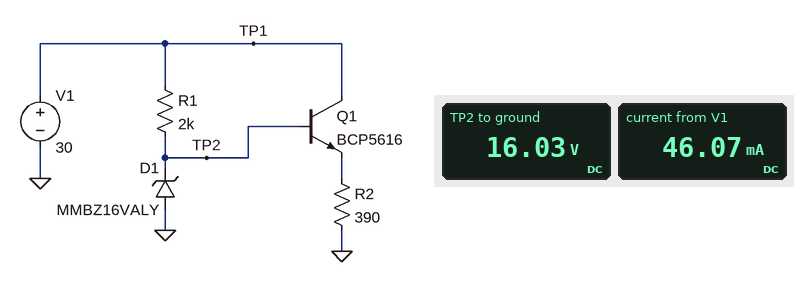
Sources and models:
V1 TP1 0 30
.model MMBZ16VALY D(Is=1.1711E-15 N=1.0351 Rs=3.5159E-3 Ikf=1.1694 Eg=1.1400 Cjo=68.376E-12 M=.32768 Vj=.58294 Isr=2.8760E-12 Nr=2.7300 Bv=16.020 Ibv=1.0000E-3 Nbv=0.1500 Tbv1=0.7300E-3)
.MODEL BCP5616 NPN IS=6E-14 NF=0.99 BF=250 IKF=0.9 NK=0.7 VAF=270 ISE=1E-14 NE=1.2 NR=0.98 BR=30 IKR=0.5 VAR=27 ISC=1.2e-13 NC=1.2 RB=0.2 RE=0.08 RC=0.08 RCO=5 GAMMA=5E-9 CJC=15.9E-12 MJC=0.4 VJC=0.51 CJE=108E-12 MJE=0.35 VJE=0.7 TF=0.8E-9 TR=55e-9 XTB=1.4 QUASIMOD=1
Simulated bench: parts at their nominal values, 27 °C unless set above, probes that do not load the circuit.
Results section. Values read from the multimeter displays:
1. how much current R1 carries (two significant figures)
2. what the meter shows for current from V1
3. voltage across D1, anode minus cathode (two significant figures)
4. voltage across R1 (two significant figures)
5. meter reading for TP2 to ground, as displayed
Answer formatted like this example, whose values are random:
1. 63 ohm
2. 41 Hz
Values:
1. 7.0 mA
2. 46.07 mA
3. -16 V
4. 14 V
5. 16.03 V
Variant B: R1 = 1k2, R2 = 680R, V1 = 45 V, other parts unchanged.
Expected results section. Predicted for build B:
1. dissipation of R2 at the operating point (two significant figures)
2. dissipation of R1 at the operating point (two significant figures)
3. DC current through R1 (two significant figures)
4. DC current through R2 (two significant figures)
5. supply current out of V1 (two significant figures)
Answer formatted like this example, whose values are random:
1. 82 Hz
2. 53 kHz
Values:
1. 350 mW
2. 700 mW
3. 24 mA
4. 23 mA
5. 47 mA
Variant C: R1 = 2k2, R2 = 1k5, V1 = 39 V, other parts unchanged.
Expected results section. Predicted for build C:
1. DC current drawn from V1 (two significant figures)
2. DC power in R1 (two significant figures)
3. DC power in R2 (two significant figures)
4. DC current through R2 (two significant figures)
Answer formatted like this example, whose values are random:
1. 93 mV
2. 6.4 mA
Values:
1. 21 mA
2. 240 mW
3. 160 mW
4. 10 mA
